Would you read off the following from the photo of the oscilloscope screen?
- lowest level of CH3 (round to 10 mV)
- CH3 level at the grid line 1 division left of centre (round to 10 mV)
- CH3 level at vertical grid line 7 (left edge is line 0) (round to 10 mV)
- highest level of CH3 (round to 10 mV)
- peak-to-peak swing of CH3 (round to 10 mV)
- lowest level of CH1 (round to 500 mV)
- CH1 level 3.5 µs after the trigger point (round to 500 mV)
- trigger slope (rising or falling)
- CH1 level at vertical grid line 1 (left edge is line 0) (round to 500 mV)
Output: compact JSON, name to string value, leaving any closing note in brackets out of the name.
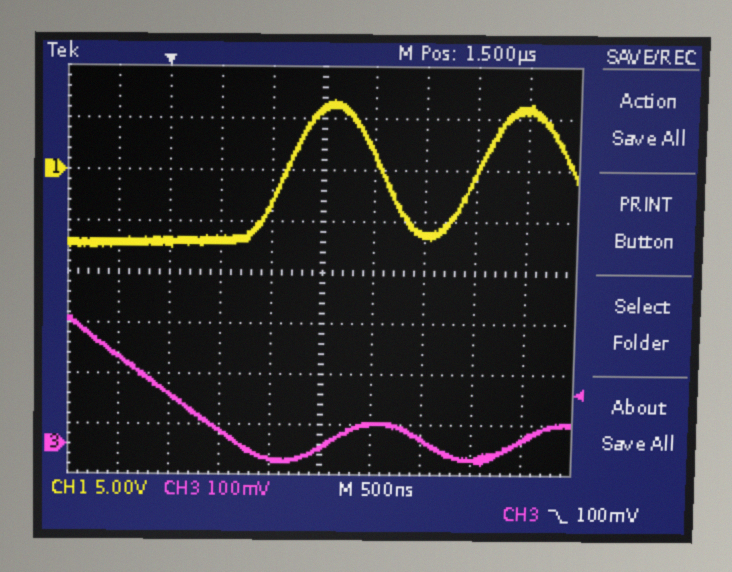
{"lowest level of CH3": "-40 mV", "CH3 level at the grid line 1 division left of centre": "-30 mV", "CH3 level at vertical grid line 7 (left edge is line 0)": "10 mV", "highest level of CH3": "250 mV", "peak-to-peak swing of CH3": "290 mV", "lowest level of CH1": "-7.5 V", "CH1 level 3.5 µs after the trigger point": "6.0 V", "trigger slope": "falling", "CH1 level at vertical grid line 1 (left edge is line 0)": "-7.0 V"}
